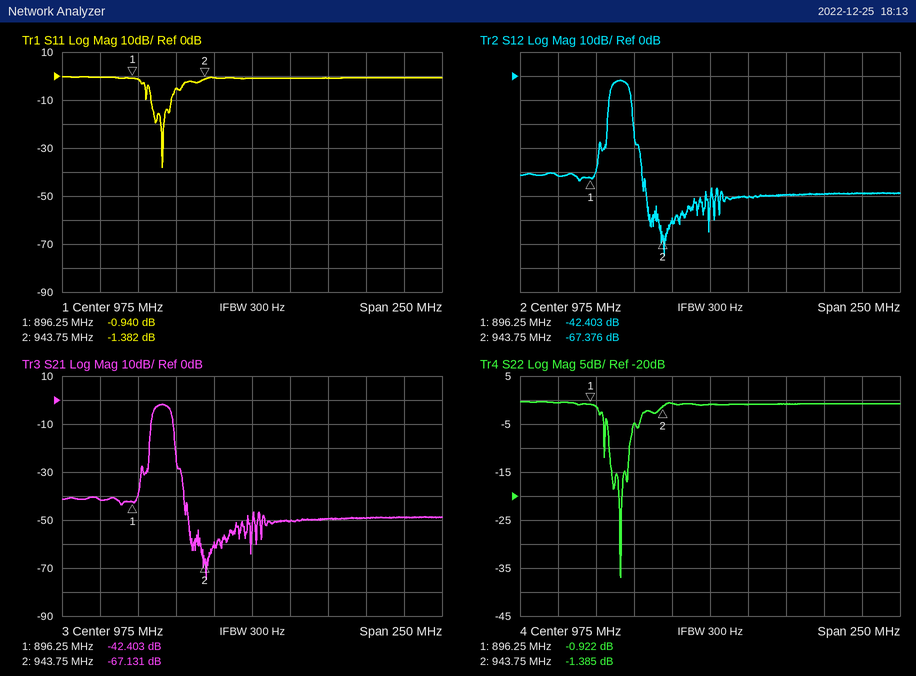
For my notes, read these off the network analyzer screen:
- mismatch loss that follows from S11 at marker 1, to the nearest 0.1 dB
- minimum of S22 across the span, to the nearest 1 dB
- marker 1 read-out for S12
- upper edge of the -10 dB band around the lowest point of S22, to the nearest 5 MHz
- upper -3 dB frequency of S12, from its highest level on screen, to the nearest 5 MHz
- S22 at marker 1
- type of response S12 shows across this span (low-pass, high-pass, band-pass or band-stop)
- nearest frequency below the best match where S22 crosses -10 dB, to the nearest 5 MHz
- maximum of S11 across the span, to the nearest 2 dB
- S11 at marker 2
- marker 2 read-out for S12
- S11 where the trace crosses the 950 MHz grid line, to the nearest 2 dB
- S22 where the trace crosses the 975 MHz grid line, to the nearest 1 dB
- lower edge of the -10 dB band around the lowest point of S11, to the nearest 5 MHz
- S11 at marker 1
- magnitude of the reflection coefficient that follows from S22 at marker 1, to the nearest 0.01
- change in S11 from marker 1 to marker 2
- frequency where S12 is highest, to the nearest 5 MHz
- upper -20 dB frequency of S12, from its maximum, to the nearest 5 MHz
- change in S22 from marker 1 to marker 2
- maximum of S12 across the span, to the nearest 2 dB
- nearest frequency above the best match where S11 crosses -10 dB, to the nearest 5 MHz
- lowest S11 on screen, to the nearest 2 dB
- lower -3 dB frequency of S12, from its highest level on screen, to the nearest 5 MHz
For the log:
7.1 dB
-37 dB
-42.403 dB
920 MHz
920 MHz
-0.922 dB
band-pass
910 MHz
0 dB
-1.382 dB
-67.376 dB
0 dB
-1 dB
910 MHz
-0.940 dB
0.90
-0.442 dB
915 MHz
925 MHz
-0.463 dB
-2 dB
920 MHz
-38 dB
910 MHz
